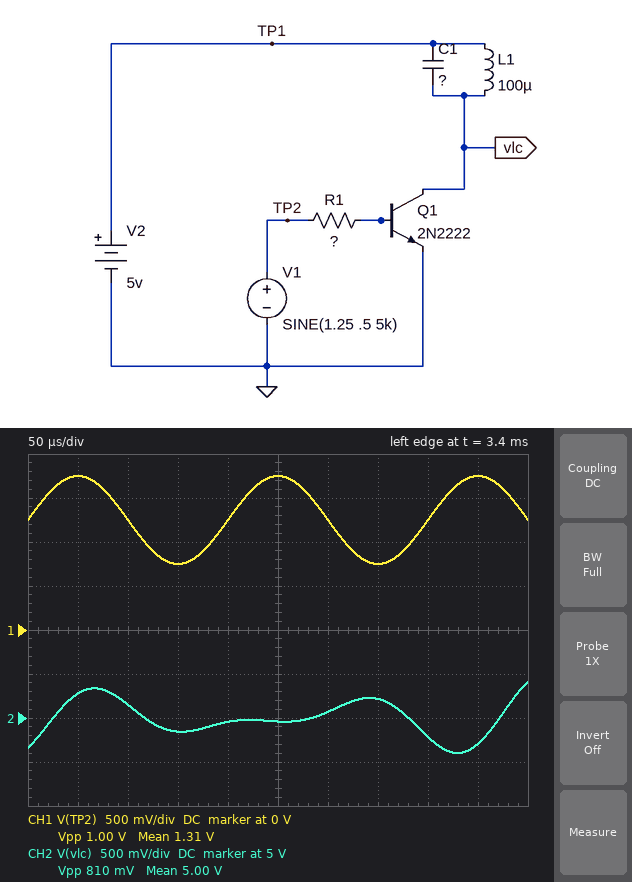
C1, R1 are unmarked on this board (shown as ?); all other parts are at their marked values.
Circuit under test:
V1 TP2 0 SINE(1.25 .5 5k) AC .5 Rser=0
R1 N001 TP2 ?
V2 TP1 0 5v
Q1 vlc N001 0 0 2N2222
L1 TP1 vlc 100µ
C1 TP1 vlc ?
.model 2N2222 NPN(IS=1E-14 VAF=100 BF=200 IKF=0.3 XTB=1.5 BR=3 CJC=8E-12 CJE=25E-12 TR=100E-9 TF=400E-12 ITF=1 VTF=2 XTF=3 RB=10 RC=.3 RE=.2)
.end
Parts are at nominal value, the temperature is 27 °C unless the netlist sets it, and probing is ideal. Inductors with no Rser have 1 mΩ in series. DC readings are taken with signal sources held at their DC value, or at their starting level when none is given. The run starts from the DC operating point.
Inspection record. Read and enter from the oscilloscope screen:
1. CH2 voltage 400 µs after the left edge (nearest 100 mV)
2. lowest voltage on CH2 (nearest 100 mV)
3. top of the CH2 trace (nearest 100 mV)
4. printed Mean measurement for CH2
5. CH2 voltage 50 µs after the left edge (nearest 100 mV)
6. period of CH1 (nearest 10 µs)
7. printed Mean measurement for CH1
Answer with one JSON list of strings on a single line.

["4.8 V", "4.6 V", "5.4 V", "5.00 V", "5.3 V", "200 µs", "1.31 V"]
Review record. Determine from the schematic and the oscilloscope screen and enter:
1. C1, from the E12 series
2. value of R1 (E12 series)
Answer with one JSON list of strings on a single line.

["6.8 µF", "2.2 kΩ"]
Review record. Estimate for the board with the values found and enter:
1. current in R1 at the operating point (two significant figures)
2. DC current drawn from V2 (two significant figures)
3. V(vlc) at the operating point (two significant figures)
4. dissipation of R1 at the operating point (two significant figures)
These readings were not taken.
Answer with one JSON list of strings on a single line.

["220 µA", "41 mA", "5.0 V", "110 µW"]
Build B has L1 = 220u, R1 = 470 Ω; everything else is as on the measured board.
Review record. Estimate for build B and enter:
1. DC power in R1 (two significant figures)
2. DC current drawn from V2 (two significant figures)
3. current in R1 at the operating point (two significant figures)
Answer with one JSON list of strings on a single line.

["380 µW", "130 mA", "900 µA"]
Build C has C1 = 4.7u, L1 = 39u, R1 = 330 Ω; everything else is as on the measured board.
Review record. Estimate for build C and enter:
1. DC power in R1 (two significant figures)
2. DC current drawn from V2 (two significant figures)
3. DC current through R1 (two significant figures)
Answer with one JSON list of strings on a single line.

["500 µW", "170 mA", "1.2 mA"]
